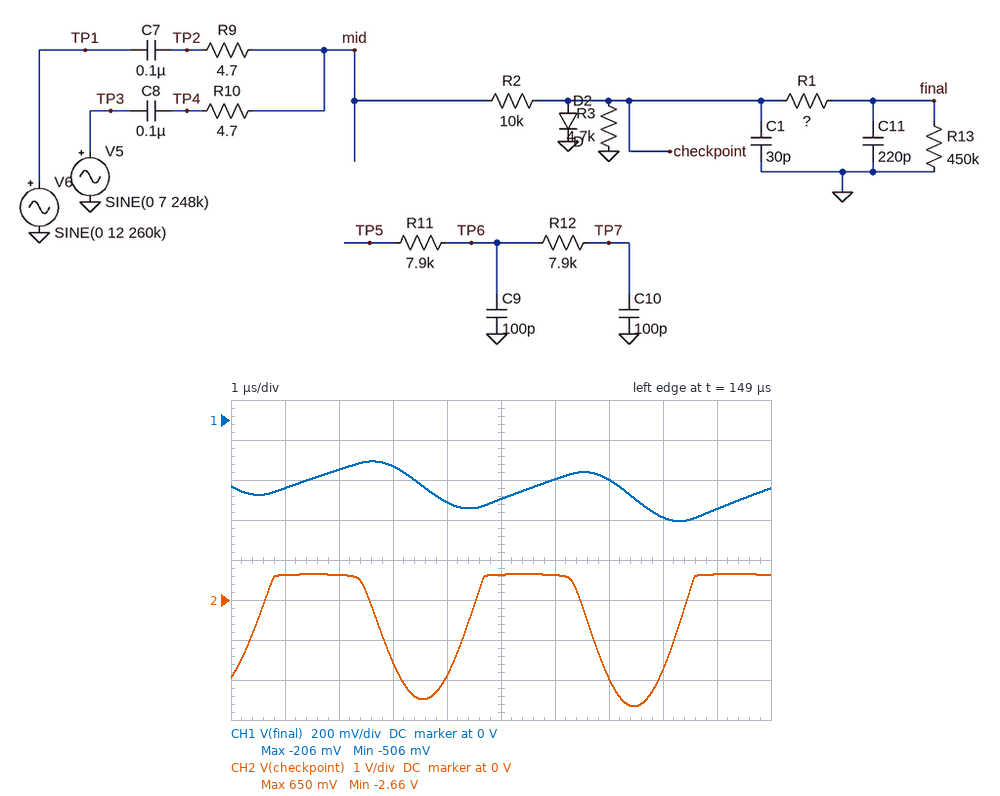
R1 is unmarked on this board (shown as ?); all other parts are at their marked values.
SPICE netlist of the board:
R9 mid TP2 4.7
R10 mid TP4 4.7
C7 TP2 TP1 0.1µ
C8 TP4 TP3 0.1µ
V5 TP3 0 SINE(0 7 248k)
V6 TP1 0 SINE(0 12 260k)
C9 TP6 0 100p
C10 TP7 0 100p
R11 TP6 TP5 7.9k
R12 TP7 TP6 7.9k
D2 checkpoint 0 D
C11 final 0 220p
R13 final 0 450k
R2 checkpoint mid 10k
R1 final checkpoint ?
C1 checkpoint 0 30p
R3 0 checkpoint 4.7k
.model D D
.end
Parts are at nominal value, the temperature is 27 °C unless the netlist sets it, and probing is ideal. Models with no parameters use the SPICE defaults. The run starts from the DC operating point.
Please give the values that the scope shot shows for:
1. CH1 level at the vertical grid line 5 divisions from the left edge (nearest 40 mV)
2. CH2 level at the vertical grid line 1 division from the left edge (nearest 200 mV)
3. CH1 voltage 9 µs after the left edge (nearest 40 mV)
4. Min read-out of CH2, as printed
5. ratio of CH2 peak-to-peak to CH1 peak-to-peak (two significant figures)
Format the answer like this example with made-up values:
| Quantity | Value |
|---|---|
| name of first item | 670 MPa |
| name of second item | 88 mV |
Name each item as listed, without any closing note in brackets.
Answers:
| Quantity | Value |
|---|---|
| CH1 level at the vertical grid line 5 divisions from the left edge | -400 mV |
| CH2 level at the vertical grid line 1 division from the left edge | 600 mV |
| CH1 voltage 9 µs after the left edge | -440 mV |
| Min read-out of CH2, as printed | -2.66 V |
| ratio of CH2 peak-to-peak to CH1 peak-to-peak | 11 |
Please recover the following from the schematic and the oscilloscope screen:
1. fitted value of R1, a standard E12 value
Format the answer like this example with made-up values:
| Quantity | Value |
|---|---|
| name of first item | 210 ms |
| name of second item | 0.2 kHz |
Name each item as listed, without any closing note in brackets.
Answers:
| Quantity | Value |
|---|---|
| fitted value of R1, a standard E12 value | 47 kΩ |
